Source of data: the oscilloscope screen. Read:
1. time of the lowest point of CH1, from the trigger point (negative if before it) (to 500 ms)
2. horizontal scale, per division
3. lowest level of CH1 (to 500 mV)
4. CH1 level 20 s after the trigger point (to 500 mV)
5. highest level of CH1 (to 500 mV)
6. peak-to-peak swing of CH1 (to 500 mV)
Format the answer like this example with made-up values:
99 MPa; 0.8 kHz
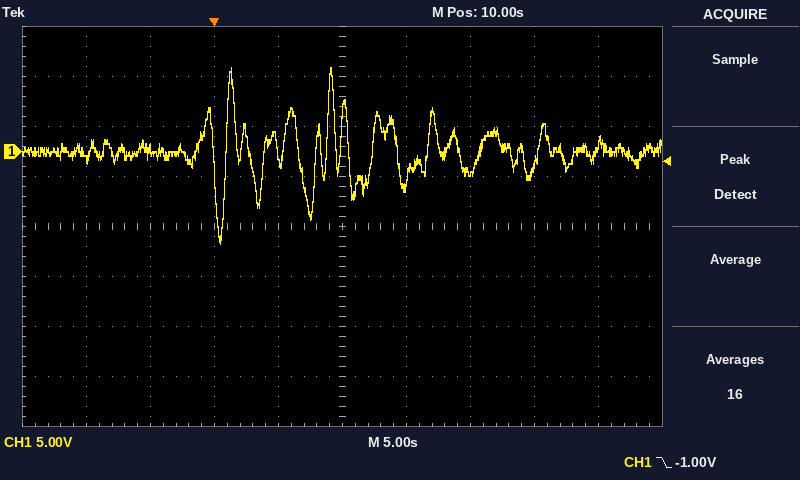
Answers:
+500 ms; 5 s; -9.0 V; -2.0 V; 8.5 V; 17.5 V
